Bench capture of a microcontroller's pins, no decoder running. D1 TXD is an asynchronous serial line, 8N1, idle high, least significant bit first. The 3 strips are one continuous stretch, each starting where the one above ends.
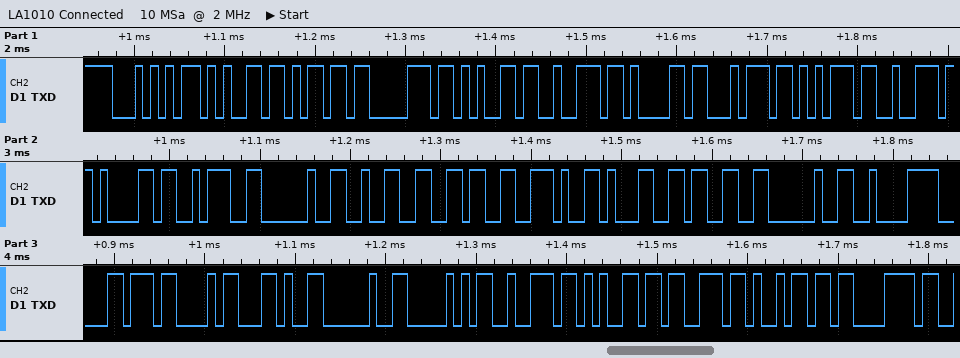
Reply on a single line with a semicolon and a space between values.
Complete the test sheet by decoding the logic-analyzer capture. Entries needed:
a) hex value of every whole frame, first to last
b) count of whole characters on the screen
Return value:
54 65 6D 70 65 72 61 74 75 72 61 3A 20 32 36 2E 31 33 20 C2 B0 43 2C 20 50 72 65 73 69 C3; 30
